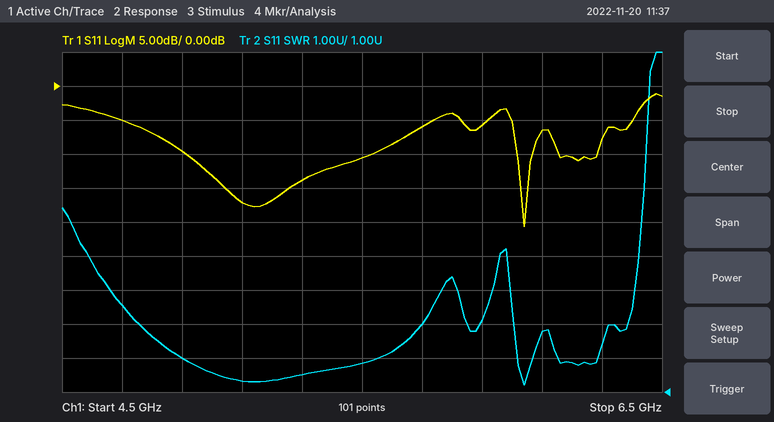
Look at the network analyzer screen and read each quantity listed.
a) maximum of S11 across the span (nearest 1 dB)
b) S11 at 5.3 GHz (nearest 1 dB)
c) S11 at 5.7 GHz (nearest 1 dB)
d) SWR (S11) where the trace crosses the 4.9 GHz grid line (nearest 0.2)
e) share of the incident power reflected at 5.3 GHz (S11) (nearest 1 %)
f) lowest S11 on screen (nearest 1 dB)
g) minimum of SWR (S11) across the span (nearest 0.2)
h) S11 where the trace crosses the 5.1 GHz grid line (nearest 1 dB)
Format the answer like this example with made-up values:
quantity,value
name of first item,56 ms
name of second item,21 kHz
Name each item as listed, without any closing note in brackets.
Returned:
quantity,value
maximum of S11 across the span,-1 dB
S11 at 5.3 GHz,-14 dB
S11 at 5.7 GHz,-6 dB
SWR (S11) where the trace crosses the 4.9 GHz grid line,2.0
share of the incident power reflected at 5.3 GHz (S11),4 %
lowest S11 on screen,-21 dB
minimum of SWR (S11) across the span,1.2
S11 where the trace crosses the 5.1 GHz grid line,-17 dB
